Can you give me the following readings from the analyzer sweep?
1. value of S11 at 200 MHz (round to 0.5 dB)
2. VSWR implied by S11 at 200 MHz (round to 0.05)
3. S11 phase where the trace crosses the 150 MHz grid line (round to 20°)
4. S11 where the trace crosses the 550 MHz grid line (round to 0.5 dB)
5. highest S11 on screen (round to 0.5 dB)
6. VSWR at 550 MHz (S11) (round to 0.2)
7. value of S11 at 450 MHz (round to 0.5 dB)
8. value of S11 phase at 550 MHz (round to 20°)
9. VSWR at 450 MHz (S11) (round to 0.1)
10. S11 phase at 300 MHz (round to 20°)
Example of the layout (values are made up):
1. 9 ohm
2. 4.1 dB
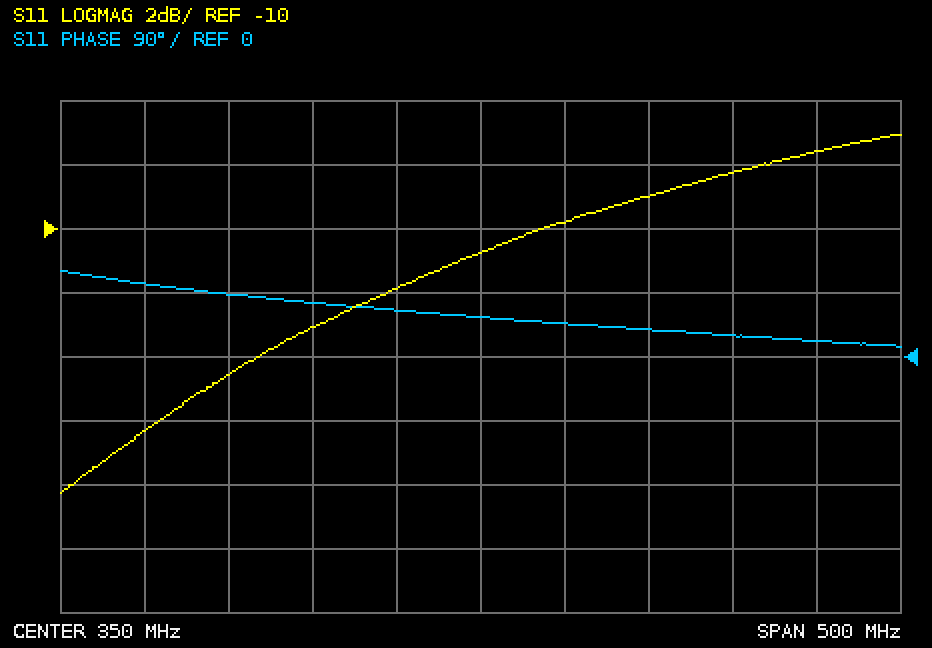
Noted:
1. -14.5 dB
2. 1.45
3. 100°
4. -7.5 dB
5. -7.0 dB
6. 2.4
7. -9.0 dB
8. 20°
9. 2.1
10. 60°
